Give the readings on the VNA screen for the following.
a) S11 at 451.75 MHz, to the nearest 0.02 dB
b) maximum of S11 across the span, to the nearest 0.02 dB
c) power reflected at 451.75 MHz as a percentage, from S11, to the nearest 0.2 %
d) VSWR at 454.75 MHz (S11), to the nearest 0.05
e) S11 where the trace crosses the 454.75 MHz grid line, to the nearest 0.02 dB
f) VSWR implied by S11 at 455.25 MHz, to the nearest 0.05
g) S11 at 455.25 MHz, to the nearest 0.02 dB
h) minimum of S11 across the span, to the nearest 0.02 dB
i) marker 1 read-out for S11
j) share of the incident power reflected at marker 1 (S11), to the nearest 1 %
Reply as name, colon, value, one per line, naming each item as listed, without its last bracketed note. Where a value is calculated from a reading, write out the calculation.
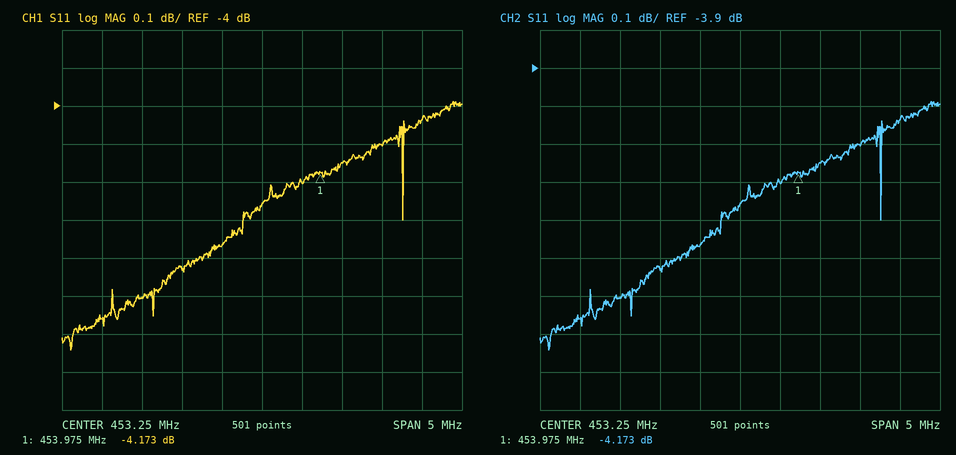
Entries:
S11 at 451.75 MHz, to the nearest 0.02 dB: -4.50 dB
maximum of S11 across the span, to the nearest 0.02 dB: -3.98 dB
power reflected at 451.75 MHz as a percentage, from S11, to the nearest 0.2 %: 10^(-4.5/10) ≈ 35.5 %, so 35.4 % to the nearest 0.2 %
VSWR at 454.75 MHz (S11), to the nearest 0.05: |Γ| = 10^(-4.1/20) = 0.6237; VSWR = (1 + 0.6237)/(1 − 0.6237) ≈ 4.32, so 4.30 to the nearest 0.05
S11 where the trace crosses the 454.75 MHz grid line, to the nearest 0.02 dB: -4.10 dB
VSWR implied by S11 at 455.25 MHz, to the nearest 0.05: |Γ| = 10^(-4.04/20) = 0.6281; VSWR = (1 + 0.6281)/(1 − 0.6281) ≈ 4.38, so 4.40 to the nearest 0.05
S11 at 455.25 MHz, to the nearest 0.02 dB: -4.04 dB
minimum of S11 across the span, to the nearest 0.02 dB: -4.64 dB
marker 1 read-out for S11: -4.173 dB
share of the incident power reflected at marker 1 (S11), to the nearest 1 %: 10^(-4.173/10) ≈ 38 %
